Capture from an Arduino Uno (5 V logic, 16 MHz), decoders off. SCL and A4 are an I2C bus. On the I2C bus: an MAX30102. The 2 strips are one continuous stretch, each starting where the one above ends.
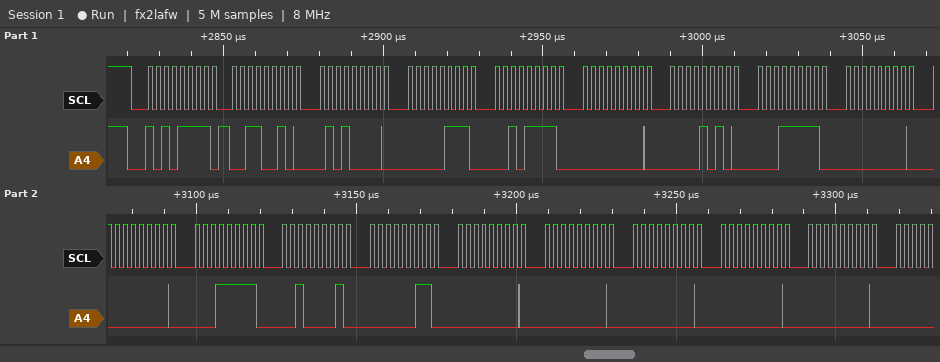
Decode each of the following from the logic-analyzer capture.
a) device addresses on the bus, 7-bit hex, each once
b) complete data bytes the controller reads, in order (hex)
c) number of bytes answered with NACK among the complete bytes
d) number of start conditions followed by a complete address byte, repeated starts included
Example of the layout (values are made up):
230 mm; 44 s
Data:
0x57; 32 50 07 2F 00 0A 1F 00 00 1F 21 03 00 00 00 00 00; 0; 1
